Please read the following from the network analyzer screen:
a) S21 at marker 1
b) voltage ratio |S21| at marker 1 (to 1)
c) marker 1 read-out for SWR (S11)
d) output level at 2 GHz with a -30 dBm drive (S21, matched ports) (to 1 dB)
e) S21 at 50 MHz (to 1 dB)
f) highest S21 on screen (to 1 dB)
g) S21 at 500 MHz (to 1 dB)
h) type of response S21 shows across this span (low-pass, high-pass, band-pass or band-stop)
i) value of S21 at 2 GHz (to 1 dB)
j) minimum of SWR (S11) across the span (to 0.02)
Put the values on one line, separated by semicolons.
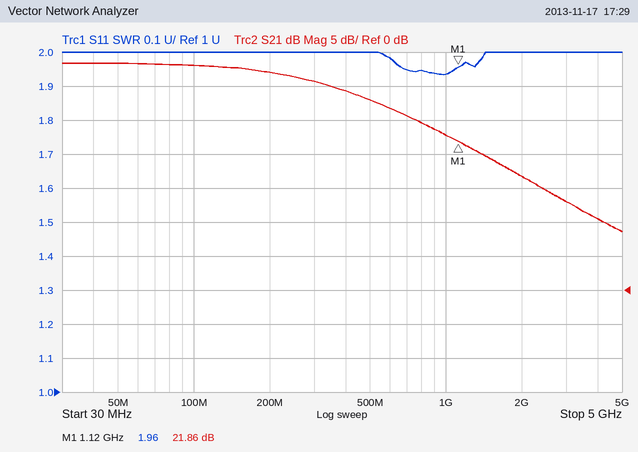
21.86 dB; 12; 1.96; -13 dBm; 33 dB; 33 dB; 28 dB; low-pass; 17 dB; 1.94
